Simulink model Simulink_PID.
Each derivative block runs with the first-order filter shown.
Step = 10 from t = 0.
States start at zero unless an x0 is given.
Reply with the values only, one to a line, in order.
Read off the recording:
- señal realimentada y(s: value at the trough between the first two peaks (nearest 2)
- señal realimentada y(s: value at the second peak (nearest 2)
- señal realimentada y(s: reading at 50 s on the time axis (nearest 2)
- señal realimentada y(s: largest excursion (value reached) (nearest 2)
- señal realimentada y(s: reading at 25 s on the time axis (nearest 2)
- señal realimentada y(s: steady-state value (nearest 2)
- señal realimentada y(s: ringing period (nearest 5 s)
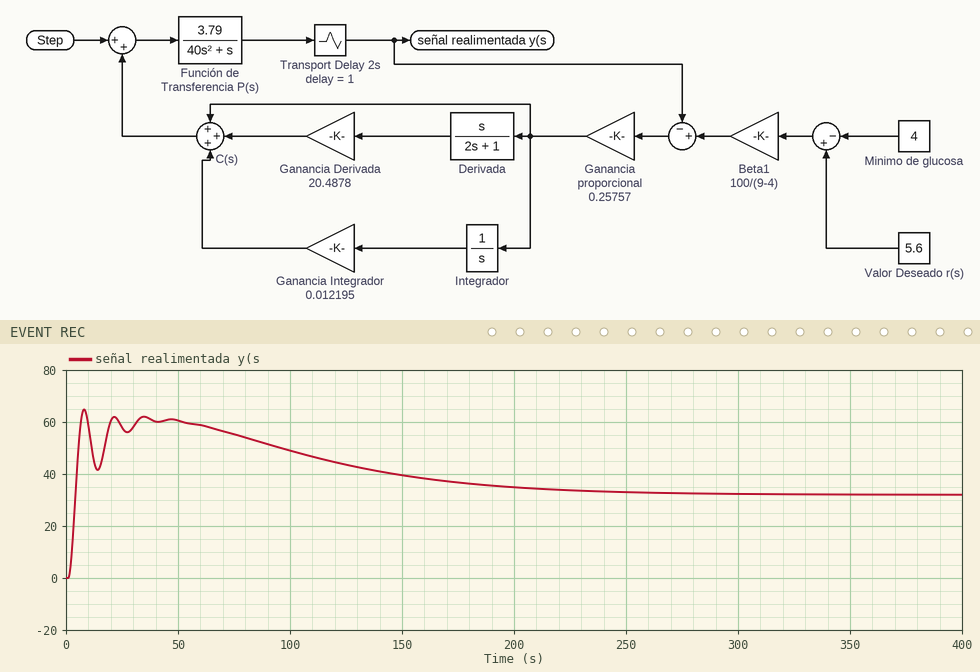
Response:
42
62
60
64
58
32
15 s
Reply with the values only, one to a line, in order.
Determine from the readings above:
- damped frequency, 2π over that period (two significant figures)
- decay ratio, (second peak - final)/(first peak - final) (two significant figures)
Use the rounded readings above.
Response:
0.42 rad/s
0.94
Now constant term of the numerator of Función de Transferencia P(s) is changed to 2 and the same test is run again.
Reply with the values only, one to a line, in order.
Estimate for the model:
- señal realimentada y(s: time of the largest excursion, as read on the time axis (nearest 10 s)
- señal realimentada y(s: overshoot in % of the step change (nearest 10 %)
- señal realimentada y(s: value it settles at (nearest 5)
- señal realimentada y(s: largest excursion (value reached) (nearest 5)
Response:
40 s
90 %
30
60
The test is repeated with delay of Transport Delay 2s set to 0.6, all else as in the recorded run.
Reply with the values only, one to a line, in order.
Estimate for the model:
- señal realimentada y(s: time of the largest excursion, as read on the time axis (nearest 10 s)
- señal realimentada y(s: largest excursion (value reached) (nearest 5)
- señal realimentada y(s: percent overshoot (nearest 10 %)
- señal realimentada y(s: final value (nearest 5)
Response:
40 s
60
90 %
30
